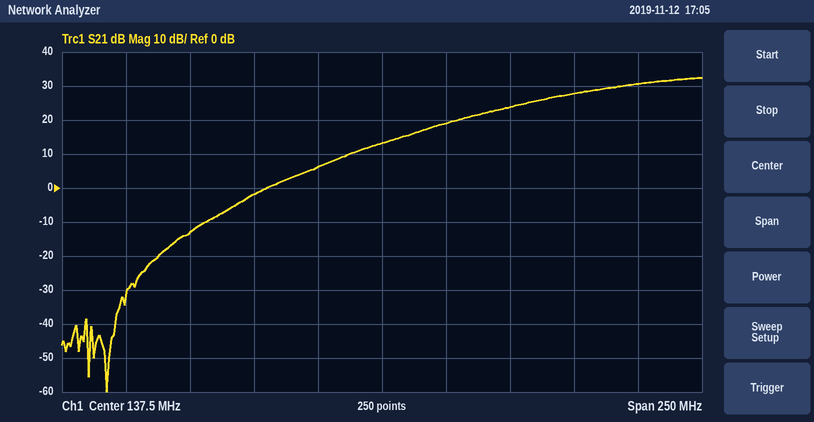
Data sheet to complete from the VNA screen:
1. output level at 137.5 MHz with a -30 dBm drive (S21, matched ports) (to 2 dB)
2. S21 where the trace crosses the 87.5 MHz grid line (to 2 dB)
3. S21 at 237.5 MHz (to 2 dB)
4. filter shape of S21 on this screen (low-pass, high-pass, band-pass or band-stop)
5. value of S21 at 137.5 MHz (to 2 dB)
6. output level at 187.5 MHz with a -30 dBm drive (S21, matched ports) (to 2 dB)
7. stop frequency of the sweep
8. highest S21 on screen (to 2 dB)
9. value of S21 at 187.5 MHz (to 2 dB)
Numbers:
-16 dBm
-2 dB
30 dB
high-pass
14 dB
-6 dBm
262.5 MHz
32 dB
24 dB
